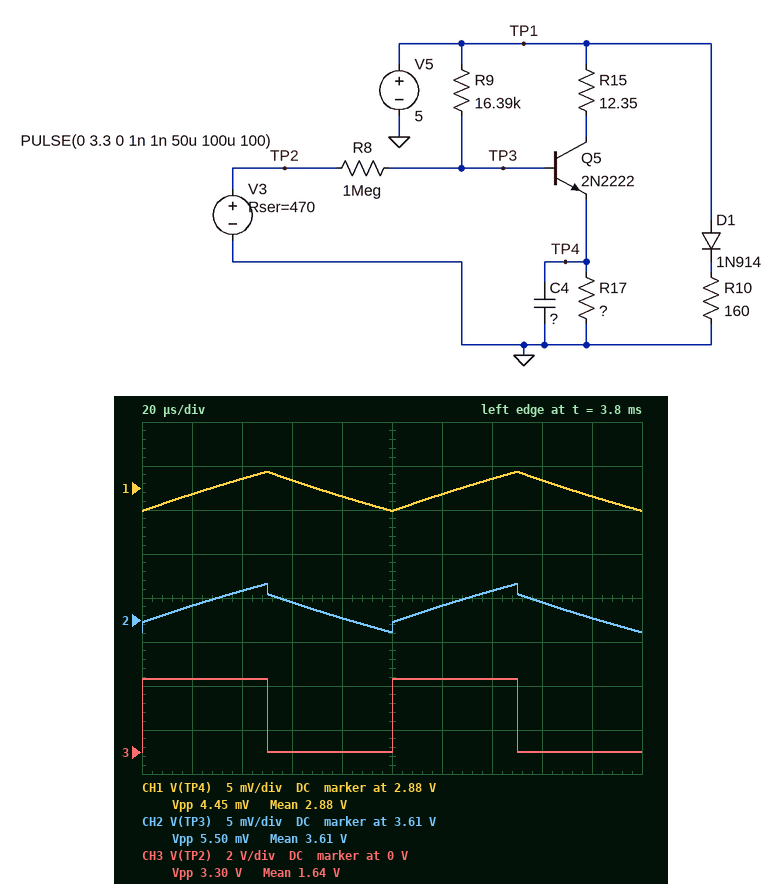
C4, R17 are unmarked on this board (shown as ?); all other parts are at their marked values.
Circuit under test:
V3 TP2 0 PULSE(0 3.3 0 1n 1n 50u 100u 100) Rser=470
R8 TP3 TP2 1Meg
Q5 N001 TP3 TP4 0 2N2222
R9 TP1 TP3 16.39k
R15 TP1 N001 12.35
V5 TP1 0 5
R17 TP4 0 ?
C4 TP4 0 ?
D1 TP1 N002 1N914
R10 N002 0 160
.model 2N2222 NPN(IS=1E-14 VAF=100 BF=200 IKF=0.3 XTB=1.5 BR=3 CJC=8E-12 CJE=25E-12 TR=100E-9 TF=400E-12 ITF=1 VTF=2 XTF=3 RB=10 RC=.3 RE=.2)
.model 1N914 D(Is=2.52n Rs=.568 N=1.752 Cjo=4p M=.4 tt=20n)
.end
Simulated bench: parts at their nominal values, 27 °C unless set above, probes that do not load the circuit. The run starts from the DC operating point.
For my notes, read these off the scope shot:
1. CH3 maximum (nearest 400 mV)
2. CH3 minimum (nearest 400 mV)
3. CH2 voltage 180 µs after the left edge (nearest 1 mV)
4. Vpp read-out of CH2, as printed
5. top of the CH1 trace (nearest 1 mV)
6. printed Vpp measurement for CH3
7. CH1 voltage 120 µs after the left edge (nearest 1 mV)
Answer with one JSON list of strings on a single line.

["3.2 V", "0 V", "3.610 V", "5.50 mV", "2.882 V", "3.30 V", "2.879 V"]
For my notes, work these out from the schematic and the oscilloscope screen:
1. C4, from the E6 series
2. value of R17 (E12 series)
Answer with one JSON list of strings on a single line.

["3.3 µF", "180 Ω"]
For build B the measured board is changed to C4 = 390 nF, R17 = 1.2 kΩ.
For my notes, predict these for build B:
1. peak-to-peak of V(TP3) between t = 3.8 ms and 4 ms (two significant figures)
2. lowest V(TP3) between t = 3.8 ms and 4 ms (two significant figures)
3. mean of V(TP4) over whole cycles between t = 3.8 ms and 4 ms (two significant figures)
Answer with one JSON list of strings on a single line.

["34 mV", "4.7 V", "4.0 V"]
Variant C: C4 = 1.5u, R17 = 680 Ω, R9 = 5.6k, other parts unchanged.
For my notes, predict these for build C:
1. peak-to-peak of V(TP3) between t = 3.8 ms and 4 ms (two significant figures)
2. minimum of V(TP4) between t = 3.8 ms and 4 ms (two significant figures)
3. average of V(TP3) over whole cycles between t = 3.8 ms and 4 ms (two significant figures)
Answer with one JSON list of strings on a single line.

["9.8 mV", "4.1 V", "4.8 V"]
